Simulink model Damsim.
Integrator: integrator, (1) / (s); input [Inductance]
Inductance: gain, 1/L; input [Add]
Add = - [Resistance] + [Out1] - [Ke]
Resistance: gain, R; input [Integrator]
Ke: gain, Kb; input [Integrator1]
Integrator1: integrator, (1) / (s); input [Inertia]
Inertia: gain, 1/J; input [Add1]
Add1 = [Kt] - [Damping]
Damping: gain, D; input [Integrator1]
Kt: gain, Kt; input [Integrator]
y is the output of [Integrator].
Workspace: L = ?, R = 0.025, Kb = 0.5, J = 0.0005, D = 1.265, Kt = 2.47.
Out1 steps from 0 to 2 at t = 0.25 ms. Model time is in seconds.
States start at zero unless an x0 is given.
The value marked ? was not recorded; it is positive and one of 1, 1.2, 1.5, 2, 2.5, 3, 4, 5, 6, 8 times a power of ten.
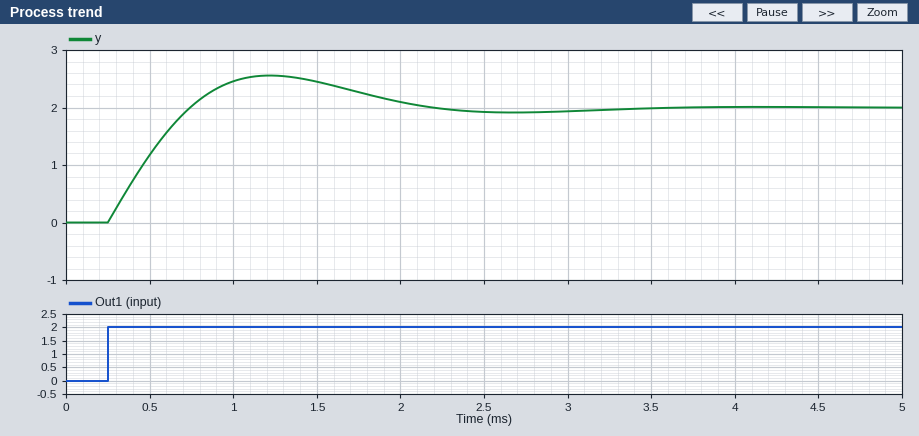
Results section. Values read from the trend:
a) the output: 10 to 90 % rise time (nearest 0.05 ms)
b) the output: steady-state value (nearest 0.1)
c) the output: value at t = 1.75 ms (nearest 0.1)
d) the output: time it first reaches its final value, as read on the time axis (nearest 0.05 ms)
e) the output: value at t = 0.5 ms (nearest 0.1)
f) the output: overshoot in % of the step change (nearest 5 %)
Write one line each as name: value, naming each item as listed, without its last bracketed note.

the output: 10 to 90 % rise time: 0.40 ms
the output: steady-state value: 2.0
the output: value at t = 1.75 ms: 2.3
the output: time it first reaches its final value, as read on the time axis: 0.75 ms
the output: value at t = 0.5 ms: 1.2
the output: overshoot in % of the step change: 30 %
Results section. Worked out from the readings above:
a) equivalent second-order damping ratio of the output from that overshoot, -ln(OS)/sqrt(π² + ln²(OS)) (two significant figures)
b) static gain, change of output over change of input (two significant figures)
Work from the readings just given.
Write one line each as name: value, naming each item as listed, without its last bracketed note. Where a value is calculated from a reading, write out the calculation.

equivalent second-order damping ratio of the output from that overshoot, -ln(OS)/sqrt(π² + ln²(OS)): ln(0.3) = -1.204; 1.204 / sqrt(9.870 + 1.450) = 0.36
static gain, change of output over change of input: (2 - 0) / (2 - 0) = 1.0
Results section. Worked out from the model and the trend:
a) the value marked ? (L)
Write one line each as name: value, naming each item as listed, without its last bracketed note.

the value marked ?: 0.0004
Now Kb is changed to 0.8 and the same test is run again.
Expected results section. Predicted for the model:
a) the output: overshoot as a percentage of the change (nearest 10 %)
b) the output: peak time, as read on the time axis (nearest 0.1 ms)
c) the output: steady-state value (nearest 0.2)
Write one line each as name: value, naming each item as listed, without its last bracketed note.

the output: overshoot as a percentage of the change: 50 %
the output: peak time, as read on the time axis: 0.9 ms
the output: steady-state value: 1.2
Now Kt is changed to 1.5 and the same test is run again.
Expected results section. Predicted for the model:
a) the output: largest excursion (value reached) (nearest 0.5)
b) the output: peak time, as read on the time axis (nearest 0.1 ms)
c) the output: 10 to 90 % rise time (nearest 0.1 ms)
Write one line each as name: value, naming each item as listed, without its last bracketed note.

the output: largest excursion (value reached): 3.5
the output: peak time, as read on the time axis: 1.8 ms
the output: 10 to 90 % rise time: 0.7 ms
